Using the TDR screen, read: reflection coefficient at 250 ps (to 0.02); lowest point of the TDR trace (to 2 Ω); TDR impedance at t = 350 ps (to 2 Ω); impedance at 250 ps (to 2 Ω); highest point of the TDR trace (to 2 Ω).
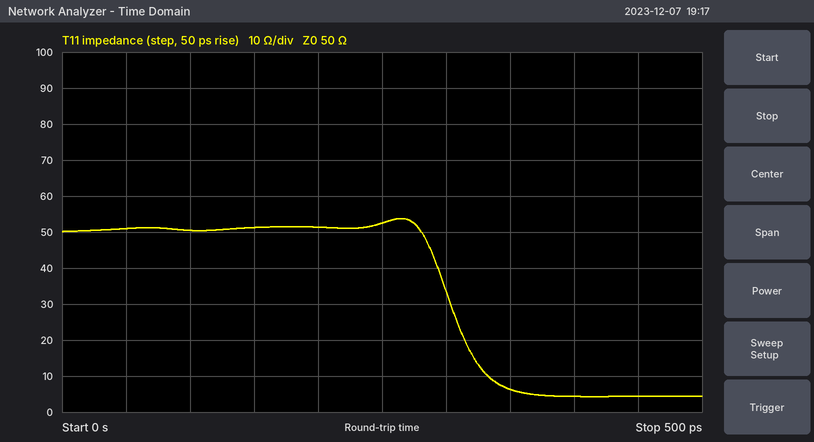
+0.02
4 Ω
6 Ω
52 Ω
54 Ω
